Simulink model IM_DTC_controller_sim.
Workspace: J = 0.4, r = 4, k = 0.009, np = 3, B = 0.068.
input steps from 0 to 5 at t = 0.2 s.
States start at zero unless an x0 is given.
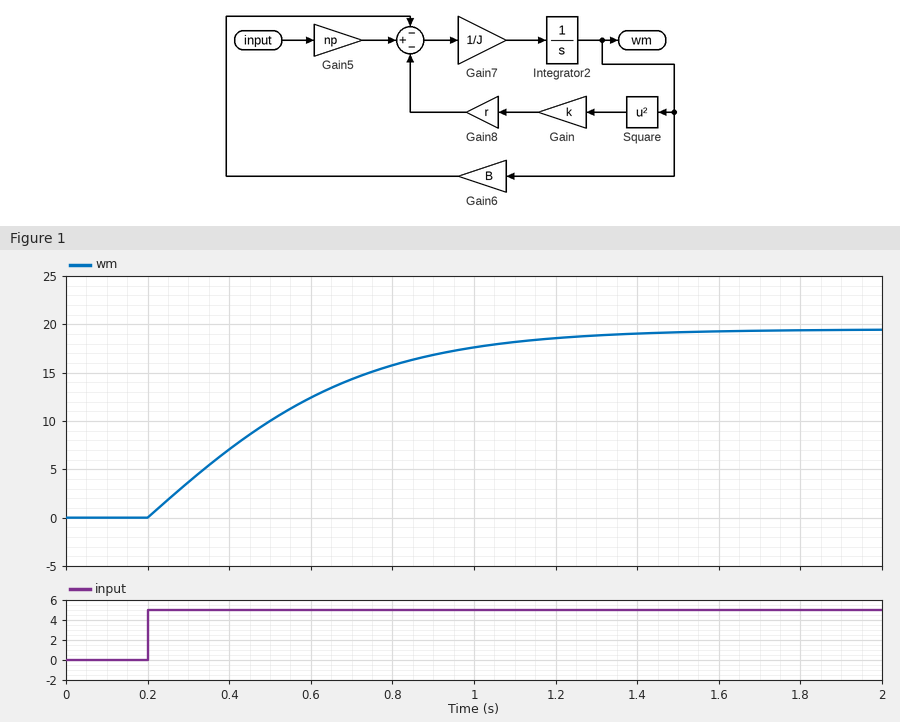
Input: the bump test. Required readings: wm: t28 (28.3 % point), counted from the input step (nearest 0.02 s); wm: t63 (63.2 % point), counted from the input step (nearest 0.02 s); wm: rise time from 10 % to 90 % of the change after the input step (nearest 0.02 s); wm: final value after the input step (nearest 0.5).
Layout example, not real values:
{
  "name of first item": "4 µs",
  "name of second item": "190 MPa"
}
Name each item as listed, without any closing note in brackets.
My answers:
{
  "wm: t28 (28.3 % point), counted from the input step": "0.16 s",
  "wm: t63 (63.2 % point), counted from the input step": "0.40 s",
  "wm: rise time from 10 % to 90 % of the change after the input step": "0.74 s",
  "wm: final value after the input step": "19.5"
}
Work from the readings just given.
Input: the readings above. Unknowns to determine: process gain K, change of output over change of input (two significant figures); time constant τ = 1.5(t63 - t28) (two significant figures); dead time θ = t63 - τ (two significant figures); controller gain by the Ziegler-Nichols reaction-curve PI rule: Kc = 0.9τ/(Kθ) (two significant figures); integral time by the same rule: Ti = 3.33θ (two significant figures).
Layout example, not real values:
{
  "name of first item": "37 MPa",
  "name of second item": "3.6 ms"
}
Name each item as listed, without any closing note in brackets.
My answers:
{
  "process gain K, change of output over change of input": "3.9",
  "time constant τ = 1.5(t63 - t28)": "0.36 s",
  "dead time θ = t63 - τ": "0.040 s",
  "controller gain by the Ziegler-Nichols reaction-curve PI rule: Kc = 0.9τ/(Kθ)": "2.1",
  "integral time by the same rule: Ti = 3.33θ": "0.13 s"
}
